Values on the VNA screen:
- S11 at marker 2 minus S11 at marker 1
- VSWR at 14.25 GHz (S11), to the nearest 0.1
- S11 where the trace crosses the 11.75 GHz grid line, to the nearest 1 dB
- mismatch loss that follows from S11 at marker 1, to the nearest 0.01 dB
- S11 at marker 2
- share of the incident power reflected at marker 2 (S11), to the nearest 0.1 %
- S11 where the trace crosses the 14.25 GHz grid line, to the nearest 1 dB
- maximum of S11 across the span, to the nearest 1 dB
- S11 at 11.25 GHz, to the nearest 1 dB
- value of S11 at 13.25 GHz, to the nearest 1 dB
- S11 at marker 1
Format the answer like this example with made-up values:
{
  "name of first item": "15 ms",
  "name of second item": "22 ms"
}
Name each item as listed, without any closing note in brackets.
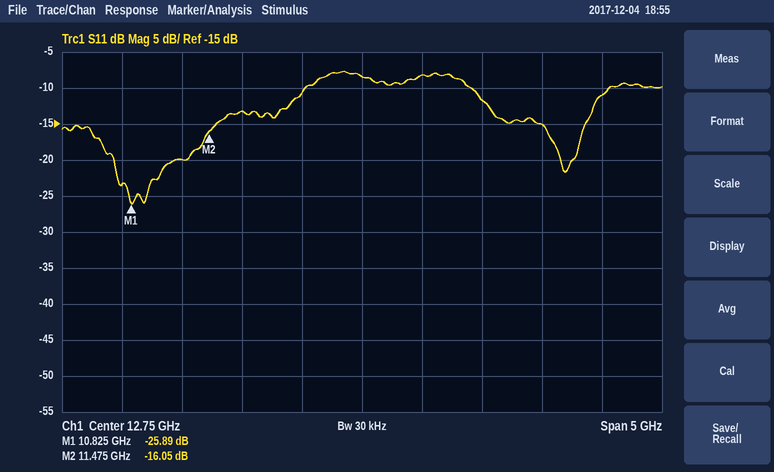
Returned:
{
  "S11 at marker 2 minus S11 at marker 1": "9.84 dB",
  "VSWR at 14.25 GHz (S11), to the nearest 0.1": "1.4",
  "S11 where the trace crosses the 11.75 GHz grid line, to the nearest 1 dB": "-13 dB",
  "mismatch loss that follows from S11 at marker 1, to the nearest 0.01 dB": "0.01 dB",
  "S11 at marker 2": "-16.05 dB",
  "share of the incident power reflected at marker 2 (S11), to the nearest 0.1 %": "2.5 %",
  "S11 where the trace crosses the 14.25 GHz grid line, to the nearest 1 dB": "-15 dB",
  "maximum of S11 across the span, to the nearest 1 dB": "-8 dB",
  "S11 at 11.25 GHz, to the nearest 1 dB": "-20 dB",
  "value of S11 at 13.25 GHz, to the nearest 1 dB": "-8 dB",
  "S11 at marker 1": "-25.89 dB"
}
